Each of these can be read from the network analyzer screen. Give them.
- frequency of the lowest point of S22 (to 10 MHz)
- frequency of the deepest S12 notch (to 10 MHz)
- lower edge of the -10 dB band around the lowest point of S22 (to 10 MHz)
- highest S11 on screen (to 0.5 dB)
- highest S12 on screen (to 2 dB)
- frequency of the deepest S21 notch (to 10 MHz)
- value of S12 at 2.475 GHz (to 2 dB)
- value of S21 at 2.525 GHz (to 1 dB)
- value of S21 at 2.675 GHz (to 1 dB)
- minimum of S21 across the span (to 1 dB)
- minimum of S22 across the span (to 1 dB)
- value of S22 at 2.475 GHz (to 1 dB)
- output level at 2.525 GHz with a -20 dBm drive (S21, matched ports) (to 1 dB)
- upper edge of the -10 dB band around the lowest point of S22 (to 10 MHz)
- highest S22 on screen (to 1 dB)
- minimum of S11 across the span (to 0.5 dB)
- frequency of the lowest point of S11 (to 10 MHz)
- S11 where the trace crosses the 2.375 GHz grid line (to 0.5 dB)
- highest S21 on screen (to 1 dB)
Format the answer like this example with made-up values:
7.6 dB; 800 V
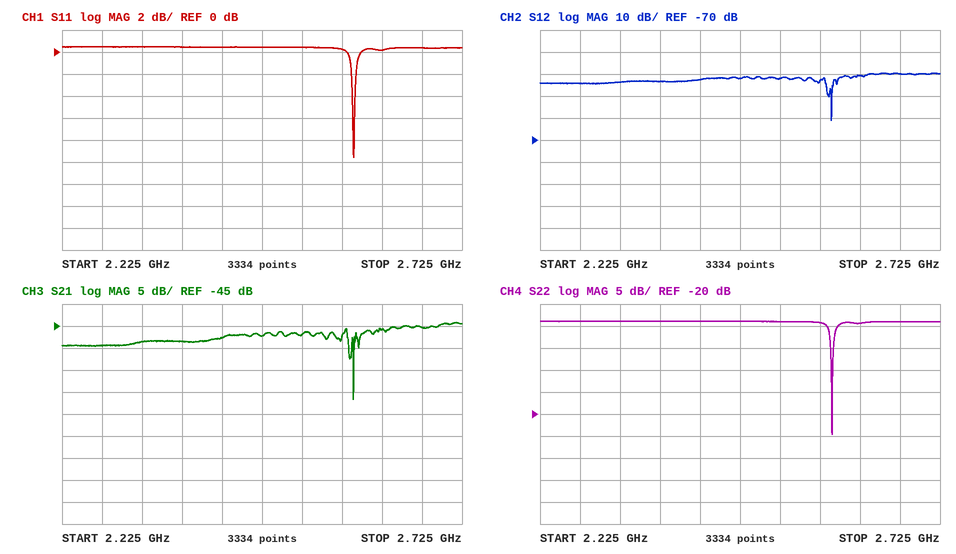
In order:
2.59 GHz; 2.59 GHz; 2.59 GHz; 0.5 dB; -40 dB; 2.59 GHz; -42 dB; -47 dB; -45 dB; -62 dB; -25 dB; 1 dB; -67 dBm; 2.59 GHz; 1 dB; -9.5 dB; 2.59 GHz; 0.5 dB; -44 dB
